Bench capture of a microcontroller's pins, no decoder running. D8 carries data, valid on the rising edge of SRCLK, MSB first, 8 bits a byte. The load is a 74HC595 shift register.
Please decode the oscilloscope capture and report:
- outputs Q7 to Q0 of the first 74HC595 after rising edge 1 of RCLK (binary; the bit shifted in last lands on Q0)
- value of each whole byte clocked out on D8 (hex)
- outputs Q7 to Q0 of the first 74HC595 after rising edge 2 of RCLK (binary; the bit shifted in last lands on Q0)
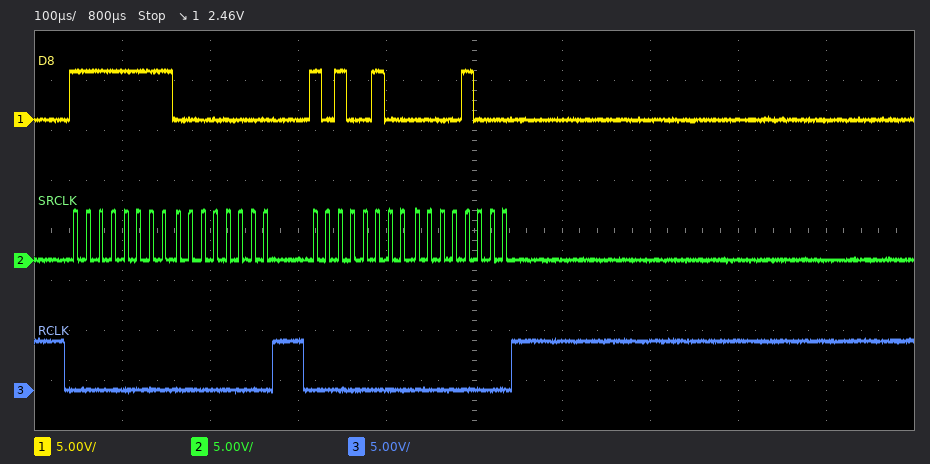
00000000
FF 00 A4 08
00001000
